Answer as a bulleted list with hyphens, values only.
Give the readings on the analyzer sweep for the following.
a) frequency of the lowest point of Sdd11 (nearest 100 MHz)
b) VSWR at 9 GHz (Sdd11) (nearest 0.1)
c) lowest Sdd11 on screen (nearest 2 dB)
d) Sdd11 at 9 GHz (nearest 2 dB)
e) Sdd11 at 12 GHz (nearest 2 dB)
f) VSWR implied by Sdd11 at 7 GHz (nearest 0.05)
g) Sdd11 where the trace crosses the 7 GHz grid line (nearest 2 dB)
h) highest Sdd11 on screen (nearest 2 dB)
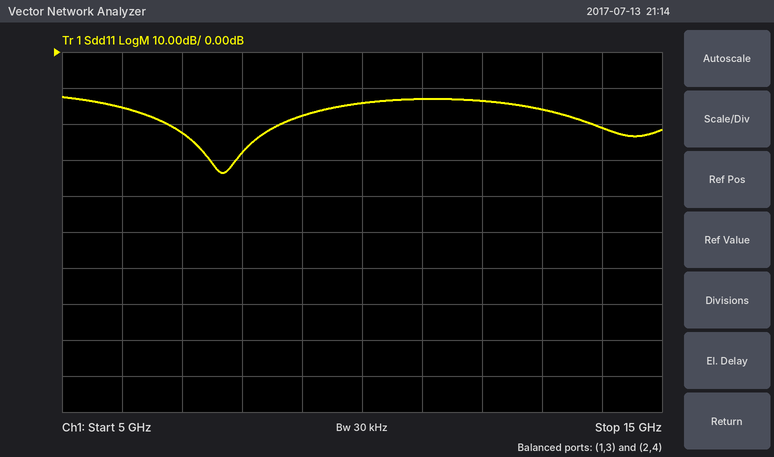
- 7.7 GHz
- 1.3
- -34 dB
- -18 dB
- -14 dB
- 1.15
- -22 dB
- -12 dB
